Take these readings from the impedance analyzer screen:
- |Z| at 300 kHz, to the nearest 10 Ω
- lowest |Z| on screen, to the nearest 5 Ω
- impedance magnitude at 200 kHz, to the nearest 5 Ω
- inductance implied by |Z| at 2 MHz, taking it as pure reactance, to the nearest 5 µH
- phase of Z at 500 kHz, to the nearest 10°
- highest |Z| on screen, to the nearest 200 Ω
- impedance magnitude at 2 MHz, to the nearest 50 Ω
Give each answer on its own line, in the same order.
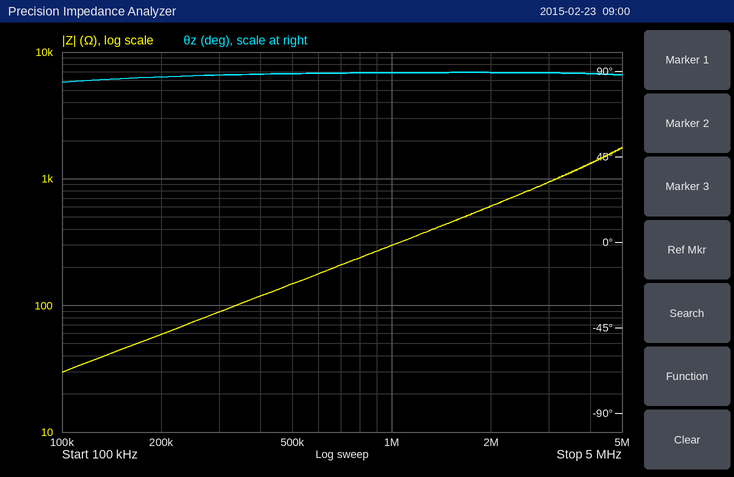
90 Ω
30 Ω
60 Ω
50 µH
90°
1.8 kΩ
600 Ω
